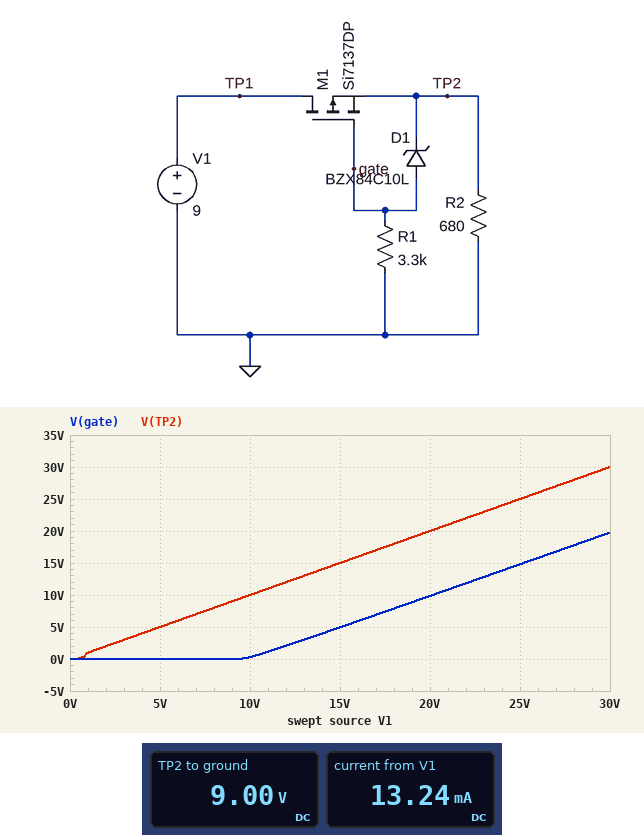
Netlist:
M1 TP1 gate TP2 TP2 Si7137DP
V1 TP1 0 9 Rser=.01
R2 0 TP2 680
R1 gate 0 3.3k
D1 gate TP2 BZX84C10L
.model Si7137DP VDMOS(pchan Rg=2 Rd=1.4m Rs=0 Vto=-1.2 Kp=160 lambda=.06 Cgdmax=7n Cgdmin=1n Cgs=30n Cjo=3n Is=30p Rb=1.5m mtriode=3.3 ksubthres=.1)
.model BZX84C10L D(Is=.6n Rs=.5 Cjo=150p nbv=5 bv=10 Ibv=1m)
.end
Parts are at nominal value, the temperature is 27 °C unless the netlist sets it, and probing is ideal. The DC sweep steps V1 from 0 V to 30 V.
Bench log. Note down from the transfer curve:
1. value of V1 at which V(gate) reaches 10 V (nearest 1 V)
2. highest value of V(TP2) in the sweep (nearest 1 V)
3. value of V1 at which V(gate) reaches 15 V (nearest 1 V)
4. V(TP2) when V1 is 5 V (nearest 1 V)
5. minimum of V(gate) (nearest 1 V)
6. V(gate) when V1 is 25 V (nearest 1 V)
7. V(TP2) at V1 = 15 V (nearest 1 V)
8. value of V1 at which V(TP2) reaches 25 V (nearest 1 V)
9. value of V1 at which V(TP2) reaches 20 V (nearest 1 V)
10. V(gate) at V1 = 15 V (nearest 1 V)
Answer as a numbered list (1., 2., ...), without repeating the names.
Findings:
1. 20 V
2. 30 V
3. 25 V
4. 5 V
5. 0 V
6. 15 V
7. 15 V
8. 25 V
9. 20 V
10. 5 V
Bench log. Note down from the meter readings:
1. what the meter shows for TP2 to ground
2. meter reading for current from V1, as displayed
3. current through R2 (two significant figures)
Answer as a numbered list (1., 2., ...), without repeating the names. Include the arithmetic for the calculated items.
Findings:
1. 9.00 V
2. 13.24 mA
3. (9 V) / 680 Ω = 13 mA
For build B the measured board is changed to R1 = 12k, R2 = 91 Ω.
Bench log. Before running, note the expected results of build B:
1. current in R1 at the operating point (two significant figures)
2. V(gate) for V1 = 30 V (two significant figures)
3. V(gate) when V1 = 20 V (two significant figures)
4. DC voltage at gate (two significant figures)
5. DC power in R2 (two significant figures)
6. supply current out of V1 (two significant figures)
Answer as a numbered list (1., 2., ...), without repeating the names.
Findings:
1. 420 nA
2. 20 V
3. 10 V
4. 5.0 mV
5. 890 mW
6. 99 mA
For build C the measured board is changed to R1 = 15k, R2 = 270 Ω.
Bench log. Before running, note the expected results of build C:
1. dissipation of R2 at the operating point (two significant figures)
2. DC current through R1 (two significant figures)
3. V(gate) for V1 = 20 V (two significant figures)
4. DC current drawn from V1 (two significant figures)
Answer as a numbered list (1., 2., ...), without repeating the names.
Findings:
1. 300 mW
2. 420 nA
3. 10 V
4. 33 mA
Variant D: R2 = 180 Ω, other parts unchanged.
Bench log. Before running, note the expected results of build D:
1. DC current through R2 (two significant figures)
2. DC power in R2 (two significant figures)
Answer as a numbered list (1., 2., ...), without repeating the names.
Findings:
1. 50 mA
2. 450 mW
